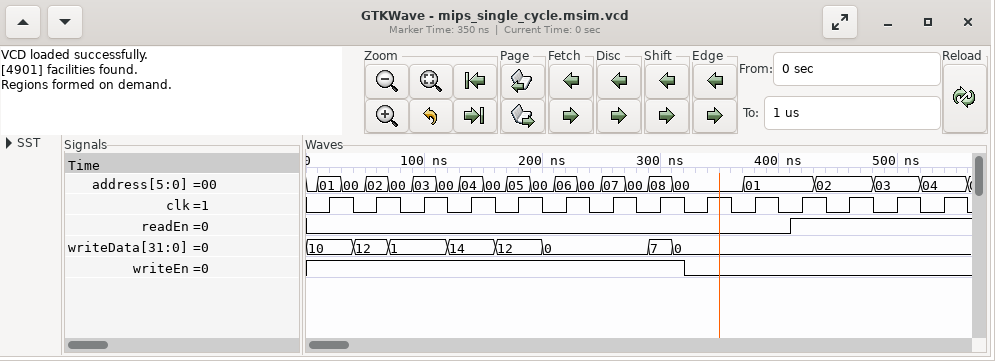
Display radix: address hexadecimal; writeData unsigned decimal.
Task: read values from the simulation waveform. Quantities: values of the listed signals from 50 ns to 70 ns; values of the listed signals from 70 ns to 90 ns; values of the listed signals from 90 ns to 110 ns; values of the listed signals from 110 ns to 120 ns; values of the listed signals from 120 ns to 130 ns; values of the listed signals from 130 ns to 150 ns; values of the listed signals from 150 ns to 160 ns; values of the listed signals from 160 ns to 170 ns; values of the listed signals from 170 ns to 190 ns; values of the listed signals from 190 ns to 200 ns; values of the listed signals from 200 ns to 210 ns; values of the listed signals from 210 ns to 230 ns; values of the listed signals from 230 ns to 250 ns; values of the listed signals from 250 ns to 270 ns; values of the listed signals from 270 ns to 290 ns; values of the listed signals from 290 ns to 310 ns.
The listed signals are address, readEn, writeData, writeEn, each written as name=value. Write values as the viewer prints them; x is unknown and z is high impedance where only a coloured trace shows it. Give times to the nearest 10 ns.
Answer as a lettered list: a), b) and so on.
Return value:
a) address=02, readEn=0, writeData=12, writeEn=1
b) address=00, readEn=0, writeData=1, writeEn=1
c) address=03, readEn=0, writeData=1, writeEn=1
d) address=00, readEn=0, writeData=1, writeEn=1
e) address=00, readEn=0, writeData=14, writeEn=1
f) address=04, readEn=0, writeData=14, writeEn=1
g) address=00, readEn=0, writeData=14, writeEn=1
h) address=00, readEn=0, writeData=12, writeEn=1
i) address=05, readEn=0, writeData=12, writeEn=1
j) address=00, readEn=0, writeData=12, writeEn=1
k) address=00, readEn=0, writeData=0, writeEn=1
l) address=06, readEn=0, writeData=0, writeEn=1
m) address=00, readEn=0, writeData=0, writeEn=1
n) address=07, readEn=0, writeData=0, writeEn=1
o) address=00, readEn=0, writeData=0, writeEn=1
p) address=08, readEn=0, writeData=7, writeEn=1
